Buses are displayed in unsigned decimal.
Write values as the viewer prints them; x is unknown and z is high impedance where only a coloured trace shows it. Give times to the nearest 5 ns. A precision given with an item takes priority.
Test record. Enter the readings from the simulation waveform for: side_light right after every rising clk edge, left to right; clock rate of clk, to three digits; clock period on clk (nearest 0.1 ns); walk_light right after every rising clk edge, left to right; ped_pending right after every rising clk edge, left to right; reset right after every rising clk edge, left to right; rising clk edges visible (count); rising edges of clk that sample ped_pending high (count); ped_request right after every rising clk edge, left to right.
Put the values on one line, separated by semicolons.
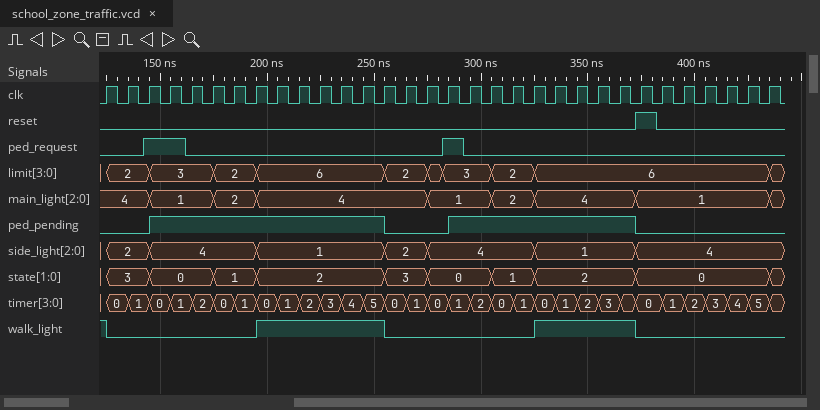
2, 2, 4, 4, 4, 4, 4, 1, 1, 1, 1, 1, 1, 2, 2, 4, 4, 4, 4, 4, 1, 1, 1, 1, 1, 4, 4, 4, 4, 4, 4, 4; 100 MHz; 10 ns; 0 0 0 0 0 0 0 1 1 1 1 1 1 0 0 0 0 0 0 0 1 1 1 1 1 0 0 0 0 0 0 0; 0 0 1 1 1 1 1 1 1 1 1 1 1 0 0 0 1 1 1 1 1 1 1 1 1 0 0 0 0 0 0 0; 0 0 0 0 0 0 0 0 0 0 0 0 0 0 0 0 0 0 0 0 0 0 0 0 0 1 0 0 0 0 0 0; 32; 19; 0 0 1 1 0 0 0 0 0 0 0 0 0 0 0 0 1 0 0 0 0 0 0 0 0 0 0 0 0 0 0 0
